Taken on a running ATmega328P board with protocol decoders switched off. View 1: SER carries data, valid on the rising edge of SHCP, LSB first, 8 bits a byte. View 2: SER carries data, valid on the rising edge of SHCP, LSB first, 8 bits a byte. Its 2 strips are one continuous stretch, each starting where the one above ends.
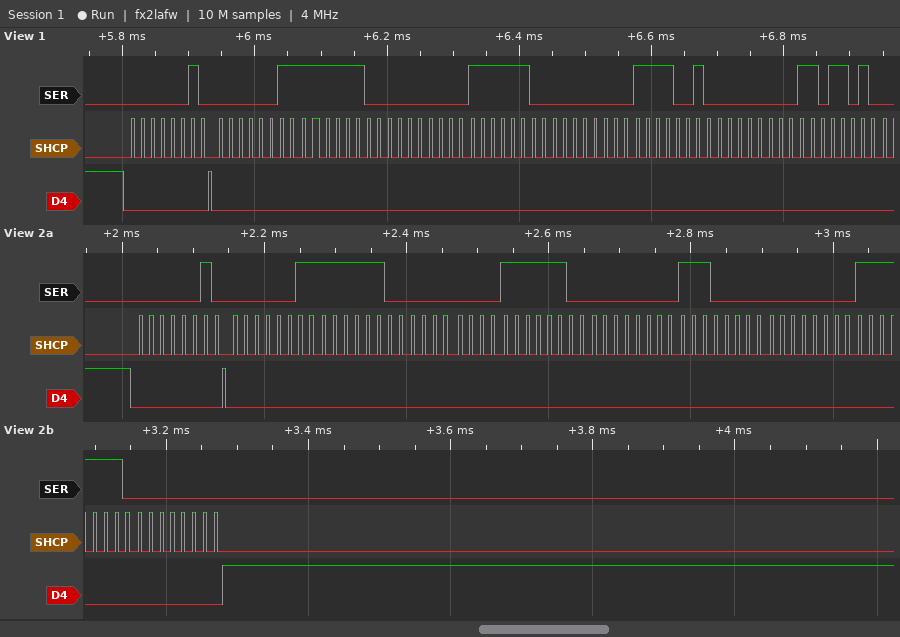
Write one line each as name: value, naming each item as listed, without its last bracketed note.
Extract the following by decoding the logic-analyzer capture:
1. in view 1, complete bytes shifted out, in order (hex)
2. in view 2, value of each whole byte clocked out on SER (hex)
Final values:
in view 1, complete bytes shifted out, in order: 40 C0 3F 00 3F 00 4F 00 5B
in view 2, value of each whole byte clocked out on SER: 40 C0 3F 00 3F 00 07 00 7F 00
